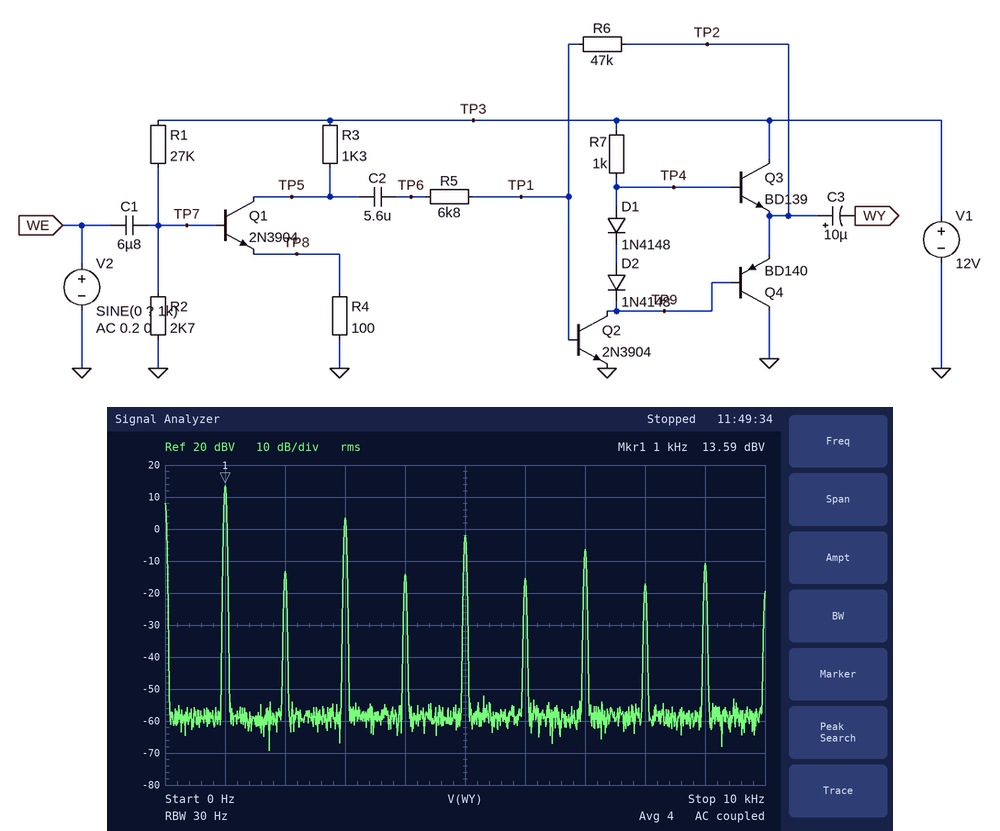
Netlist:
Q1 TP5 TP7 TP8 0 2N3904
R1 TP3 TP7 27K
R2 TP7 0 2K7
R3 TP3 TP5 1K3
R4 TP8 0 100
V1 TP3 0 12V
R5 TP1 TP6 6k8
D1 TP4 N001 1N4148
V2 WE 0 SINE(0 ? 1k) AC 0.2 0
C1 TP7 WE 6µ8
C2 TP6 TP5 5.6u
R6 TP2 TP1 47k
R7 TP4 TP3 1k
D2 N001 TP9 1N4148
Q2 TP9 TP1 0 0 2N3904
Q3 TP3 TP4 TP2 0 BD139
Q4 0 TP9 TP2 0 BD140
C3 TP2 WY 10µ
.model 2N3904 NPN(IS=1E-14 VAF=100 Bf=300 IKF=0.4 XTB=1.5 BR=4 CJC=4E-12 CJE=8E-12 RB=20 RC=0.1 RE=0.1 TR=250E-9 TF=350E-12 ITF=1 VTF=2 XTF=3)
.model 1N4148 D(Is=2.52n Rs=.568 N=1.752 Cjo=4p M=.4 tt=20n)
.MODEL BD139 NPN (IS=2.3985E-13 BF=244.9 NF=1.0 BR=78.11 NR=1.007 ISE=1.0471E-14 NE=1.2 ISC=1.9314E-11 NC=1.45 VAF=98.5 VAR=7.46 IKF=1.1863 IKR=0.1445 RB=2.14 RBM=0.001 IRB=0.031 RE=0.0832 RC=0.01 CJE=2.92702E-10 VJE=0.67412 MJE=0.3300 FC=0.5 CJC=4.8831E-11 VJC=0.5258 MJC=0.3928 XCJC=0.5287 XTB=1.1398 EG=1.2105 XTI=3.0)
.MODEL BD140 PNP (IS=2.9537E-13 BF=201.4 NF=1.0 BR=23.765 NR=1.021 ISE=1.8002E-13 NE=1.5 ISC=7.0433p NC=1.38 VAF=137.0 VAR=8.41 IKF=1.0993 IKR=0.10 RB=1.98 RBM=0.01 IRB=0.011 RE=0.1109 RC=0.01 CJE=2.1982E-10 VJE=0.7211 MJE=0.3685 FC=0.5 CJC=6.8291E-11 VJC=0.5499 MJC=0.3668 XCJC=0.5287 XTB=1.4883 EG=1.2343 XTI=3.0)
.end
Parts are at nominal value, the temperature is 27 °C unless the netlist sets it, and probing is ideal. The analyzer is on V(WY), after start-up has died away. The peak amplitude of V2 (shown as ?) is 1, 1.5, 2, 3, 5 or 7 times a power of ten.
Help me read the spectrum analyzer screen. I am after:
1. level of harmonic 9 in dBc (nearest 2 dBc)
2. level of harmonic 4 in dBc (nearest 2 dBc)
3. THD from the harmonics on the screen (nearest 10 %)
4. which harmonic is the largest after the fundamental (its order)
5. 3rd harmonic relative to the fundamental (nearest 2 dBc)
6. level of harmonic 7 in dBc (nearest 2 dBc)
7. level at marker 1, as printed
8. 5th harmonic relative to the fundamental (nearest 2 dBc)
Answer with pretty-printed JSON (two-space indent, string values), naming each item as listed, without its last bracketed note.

{
  "level of harmonic 9 in dBc": "-24 dBc",
  "level of harmonic 4 in dBc": "-28 dBc",
  "THD from the harmonics on the screen": "40 %",
  "which harmonic is the largest after the fundamental": "3",
  "3rd harmonic relative to the fundamental": "-10 dBc",
  "level of harmonic 7 in dBc": "-20 dBc",
  "level at marker 1, as printed": "13.59 dBV",
  "5th harmonic relative to the fundamental": "-16 dBc"
}
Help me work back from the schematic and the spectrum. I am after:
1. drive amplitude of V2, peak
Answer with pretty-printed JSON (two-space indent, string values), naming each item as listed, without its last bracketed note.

{
  "drive amplitude of V2, peak": "500 mV"
}
